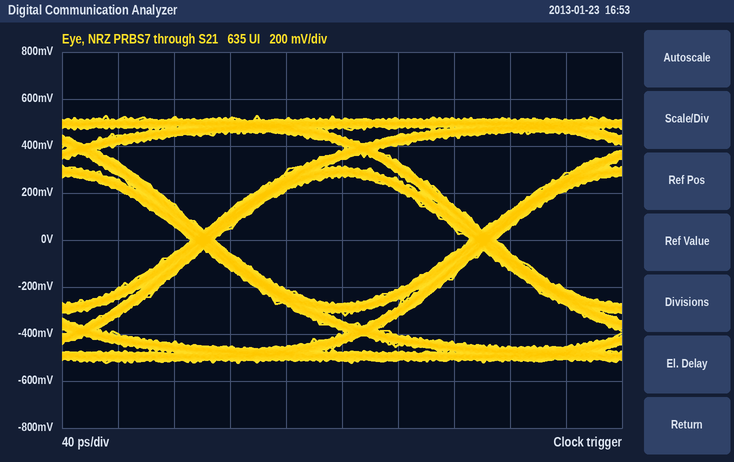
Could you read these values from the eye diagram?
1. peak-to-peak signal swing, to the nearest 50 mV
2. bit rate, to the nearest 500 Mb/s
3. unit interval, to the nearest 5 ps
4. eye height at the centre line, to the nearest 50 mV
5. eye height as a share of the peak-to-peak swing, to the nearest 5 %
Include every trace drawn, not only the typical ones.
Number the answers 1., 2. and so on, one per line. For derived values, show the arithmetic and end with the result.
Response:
1. 1.05 V
2. 5.0 Gb/s
3. 200 ps
4. 550 mV
5. 550 mV / 1.05 V ≈ 52.4 %, so 50 % to the nearest 5 %
